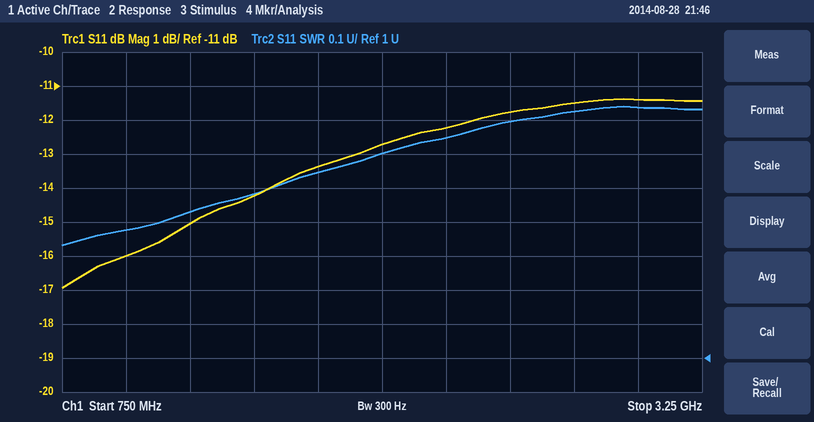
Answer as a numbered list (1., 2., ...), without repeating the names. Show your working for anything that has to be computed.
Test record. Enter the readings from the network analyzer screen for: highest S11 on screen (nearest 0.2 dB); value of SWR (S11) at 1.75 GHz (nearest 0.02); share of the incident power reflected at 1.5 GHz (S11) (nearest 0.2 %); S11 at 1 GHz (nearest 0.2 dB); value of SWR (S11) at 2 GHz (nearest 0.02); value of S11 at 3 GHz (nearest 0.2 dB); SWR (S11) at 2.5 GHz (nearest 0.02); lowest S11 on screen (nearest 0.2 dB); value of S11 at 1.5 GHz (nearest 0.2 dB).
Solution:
1. -11.4 dB
2. 1.54
3. 10^(-14.2/10) ≈ 3.8 %
4. -16.0 dB
5. 1.60
6. -11.4 dB
7. 1.70
8. -17.0 dB
9. -14.2 dB
